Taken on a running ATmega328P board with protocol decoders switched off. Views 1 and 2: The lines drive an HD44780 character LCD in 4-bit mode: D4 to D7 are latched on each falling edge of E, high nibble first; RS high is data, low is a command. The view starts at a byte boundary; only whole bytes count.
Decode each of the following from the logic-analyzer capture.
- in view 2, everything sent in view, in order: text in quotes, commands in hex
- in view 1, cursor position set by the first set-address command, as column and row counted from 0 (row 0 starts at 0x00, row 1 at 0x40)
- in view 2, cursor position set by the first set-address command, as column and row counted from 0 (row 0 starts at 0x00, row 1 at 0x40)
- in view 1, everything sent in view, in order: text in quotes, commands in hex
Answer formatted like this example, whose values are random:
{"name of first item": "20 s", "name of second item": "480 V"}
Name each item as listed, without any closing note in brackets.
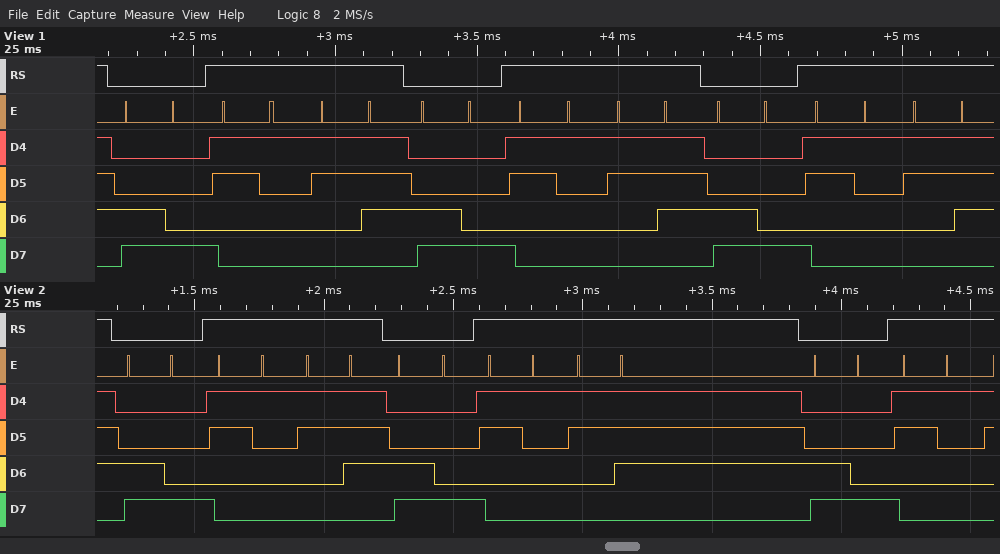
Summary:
{"in view 2, everything sent in view, in order: text in quotes, commands in hex": "0xC8 \"17\" 0xC8 \"17\" 0xC8 \"1\"", "in view 1, cursor position set by the first set-address command, as column and row counted from 0": "column 8, row 1", "in view 2, cursor position set by the first set-address command, as column and row counted from 0": "column 8, row 1", "in view 1, everything sent in view, in order: text in quotes, commands in hex": "0xC8 \"17\" 0xC8 \"17\" 0xC8 \"17\""}
